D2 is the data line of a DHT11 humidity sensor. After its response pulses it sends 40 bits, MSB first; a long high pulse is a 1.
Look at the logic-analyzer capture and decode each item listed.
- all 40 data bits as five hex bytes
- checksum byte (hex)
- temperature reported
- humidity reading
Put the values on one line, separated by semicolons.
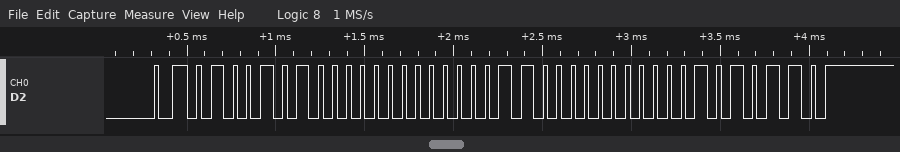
4A 00 0C 00 56; 0x56; 12.0 °C; 74 %
